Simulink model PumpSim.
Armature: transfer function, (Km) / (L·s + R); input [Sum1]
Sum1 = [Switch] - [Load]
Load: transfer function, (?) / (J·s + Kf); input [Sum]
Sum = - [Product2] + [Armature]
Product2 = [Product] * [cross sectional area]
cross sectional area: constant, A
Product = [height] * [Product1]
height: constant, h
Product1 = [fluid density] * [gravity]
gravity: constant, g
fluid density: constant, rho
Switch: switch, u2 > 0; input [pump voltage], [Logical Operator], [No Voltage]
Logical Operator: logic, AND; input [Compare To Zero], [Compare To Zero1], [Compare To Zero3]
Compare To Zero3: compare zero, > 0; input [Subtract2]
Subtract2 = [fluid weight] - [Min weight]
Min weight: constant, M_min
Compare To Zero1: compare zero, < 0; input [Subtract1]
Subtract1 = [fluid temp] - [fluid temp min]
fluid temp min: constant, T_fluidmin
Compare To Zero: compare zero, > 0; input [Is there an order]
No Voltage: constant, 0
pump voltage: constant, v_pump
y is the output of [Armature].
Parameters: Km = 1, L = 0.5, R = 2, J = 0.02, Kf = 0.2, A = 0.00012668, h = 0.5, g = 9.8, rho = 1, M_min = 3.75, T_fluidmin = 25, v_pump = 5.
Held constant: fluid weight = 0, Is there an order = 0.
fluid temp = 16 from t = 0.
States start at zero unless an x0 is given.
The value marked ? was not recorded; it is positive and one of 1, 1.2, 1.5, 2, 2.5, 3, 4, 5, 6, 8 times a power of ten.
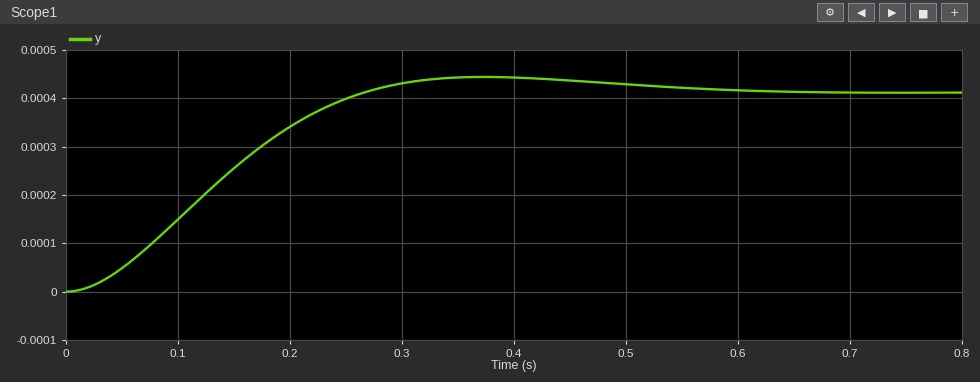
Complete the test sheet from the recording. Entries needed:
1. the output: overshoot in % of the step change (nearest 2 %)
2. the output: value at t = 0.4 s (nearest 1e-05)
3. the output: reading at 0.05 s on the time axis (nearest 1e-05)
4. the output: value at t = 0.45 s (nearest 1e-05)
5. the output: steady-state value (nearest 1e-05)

8 %
0.00044
0.00005
0.00044
0.00041
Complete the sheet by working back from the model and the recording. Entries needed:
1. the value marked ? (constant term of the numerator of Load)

0.8
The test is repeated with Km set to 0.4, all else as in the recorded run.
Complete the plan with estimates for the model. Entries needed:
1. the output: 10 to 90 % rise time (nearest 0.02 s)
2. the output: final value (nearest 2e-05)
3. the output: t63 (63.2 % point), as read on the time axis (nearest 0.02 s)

0.30 s
0.00028
0.22 s
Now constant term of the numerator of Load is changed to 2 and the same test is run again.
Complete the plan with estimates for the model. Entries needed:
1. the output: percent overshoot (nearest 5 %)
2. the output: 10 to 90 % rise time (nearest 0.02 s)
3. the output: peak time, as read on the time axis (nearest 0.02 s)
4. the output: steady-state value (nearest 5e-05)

20 %
0.10 s
0.22 s
0.00050
